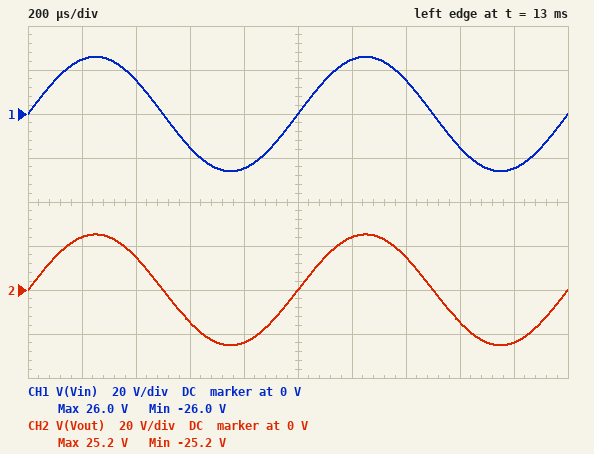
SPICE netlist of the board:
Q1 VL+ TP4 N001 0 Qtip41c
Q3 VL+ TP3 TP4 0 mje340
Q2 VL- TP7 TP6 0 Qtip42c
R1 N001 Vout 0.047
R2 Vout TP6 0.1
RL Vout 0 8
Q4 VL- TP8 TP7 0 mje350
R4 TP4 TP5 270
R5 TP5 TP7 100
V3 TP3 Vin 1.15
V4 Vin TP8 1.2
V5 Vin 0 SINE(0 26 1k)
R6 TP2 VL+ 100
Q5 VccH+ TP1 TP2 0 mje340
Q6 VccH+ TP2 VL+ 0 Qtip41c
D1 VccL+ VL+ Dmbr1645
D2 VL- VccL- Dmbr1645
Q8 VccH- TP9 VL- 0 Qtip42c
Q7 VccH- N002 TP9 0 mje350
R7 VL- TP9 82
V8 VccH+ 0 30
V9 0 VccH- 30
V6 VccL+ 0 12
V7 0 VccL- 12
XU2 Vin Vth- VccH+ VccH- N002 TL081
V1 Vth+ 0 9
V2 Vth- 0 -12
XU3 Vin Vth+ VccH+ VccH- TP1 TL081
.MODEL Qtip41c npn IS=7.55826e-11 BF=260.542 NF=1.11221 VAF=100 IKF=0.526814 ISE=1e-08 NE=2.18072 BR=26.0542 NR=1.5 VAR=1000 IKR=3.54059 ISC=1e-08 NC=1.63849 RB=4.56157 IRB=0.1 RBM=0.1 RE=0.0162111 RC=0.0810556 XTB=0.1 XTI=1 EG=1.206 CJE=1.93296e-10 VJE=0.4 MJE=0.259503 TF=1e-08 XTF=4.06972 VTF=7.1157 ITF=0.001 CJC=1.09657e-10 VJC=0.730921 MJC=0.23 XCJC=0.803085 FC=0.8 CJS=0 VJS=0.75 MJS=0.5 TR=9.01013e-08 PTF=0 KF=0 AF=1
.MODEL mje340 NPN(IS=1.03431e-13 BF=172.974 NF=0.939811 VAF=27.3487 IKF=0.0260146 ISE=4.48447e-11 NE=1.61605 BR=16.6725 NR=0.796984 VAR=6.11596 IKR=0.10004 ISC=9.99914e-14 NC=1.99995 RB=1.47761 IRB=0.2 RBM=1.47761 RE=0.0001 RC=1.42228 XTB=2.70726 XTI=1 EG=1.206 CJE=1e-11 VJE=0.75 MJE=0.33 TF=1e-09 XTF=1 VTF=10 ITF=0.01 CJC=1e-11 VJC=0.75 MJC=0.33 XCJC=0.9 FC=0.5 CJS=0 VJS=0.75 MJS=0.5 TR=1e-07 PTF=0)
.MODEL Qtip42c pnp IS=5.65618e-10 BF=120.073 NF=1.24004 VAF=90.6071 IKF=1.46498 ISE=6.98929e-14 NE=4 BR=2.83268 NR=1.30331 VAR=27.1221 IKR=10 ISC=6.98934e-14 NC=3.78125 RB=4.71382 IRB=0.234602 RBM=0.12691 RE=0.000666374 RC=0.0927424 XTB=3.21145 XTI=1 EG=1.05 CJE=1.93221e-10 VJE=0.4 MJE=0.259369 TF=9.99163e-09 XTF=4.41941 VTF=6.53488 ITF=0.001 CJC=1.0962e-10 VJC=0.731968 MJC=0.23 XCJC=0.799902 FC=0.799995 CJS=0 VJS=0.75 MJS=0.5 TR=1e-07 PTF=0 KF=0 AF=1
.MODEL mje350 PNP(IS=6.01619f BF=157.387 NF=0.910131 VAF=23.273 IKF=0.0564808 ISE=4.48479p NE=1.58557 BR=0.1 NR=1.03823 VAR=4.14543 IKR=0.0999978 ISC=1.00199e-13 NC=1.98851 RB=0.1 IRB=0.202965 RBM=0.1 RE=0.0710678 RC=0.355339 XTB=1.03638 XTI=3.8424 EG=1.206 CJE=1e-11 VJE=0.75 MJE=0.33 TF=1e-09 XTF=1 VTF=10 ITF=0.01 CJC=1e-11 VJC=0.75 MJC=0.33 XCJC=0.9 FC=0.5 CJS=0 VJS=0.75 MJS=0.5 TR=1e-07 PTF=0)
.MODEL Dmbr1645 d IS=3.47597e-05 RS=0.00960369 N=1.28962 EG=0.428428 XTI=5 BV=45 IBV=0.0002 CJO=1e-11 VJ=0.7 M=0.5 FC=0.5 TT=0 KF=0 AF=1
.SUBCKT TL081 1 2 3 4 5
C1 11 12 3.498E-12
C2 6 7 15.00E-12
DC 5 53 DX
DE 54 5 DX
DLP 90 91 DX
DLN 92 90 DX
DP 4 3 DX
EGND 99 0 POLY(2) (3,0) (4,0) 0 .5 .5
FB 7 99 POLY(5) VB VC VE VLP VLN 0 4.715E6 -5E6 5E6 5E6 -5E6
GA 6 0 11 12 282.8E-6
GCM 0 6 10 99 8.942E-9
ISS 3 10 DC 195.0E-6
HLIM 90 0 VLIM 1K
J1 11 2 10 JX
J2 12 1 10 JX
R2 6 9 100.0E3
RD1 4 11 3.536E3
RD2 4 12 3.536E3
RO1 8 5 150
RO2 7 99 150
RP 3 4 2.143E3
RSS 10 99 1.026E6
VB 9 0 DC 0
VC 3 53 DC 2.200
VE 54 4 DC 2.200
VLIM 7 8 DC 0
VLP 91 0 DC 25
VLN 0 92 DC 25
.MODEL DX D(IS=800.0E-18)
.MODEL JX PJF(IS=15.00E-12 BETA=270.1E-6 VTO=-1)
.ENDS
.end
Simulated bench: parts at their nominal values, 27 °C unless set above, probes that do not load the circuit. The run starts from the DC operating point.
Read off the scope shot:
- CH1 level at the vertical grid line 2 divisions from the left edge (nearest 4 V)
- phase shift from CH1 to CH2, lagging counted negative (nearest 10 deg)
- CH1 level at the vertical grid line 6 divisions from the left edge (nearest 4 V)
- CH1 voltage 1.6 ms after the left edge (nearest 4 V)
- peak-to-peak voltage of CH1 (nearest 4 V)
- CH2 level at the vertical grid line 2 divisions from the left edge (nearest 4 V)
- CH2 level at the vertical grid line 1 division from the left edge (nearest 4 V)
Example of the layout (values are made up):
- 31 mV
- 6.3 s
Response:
- 16 V
- 0 deg
- 24 V
- -16 V
- 52 V
- 16 V
- 24 V
